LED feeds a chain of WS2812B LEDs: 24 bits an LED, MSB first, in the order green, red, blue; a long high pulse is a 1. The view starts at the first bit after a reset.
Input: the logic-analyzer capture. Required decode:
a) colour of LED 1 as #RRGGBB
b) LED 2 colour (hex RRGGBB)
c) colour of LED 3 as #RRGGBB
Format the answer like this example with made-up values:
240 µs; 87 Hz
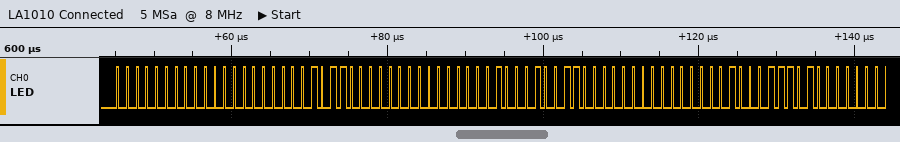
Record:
#00000B; #010013; #01001D
